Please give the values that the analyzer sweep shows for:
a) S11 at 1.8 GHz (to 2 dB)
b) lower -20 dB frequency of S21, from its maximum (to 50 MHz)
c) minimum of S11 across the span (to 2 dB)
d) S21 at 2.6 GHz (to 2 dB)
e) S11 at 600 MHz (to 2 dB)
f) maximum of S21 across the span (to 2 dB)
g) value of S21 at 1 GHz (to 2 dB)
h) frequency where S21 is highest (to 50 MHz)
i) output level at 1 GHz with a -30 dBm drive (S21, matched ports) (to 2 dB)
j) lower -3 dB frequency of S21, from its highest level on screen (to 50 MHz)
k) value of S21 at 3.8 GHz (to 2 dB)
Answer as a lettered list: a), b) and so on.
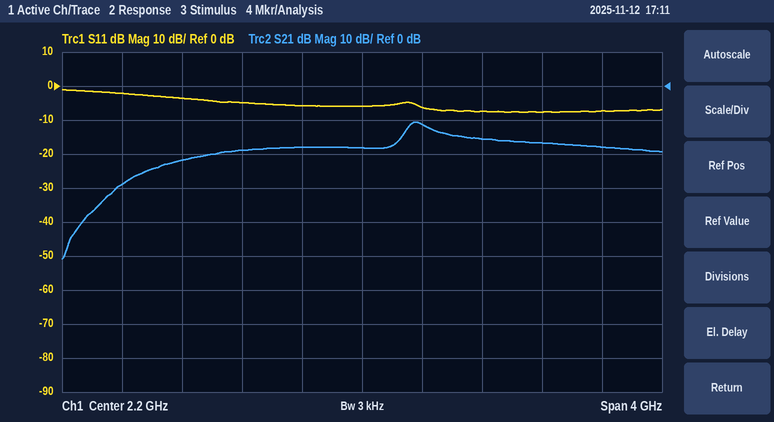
a) -6 dB
b) 550 MHz
c) -8 dB
d) -12 dB
e) -2 dB
f) -10 dB
g) -22 dB
h) 2.55 GHz
i) -52 dBm
j) 2.50 GHz
k) -18 dB
